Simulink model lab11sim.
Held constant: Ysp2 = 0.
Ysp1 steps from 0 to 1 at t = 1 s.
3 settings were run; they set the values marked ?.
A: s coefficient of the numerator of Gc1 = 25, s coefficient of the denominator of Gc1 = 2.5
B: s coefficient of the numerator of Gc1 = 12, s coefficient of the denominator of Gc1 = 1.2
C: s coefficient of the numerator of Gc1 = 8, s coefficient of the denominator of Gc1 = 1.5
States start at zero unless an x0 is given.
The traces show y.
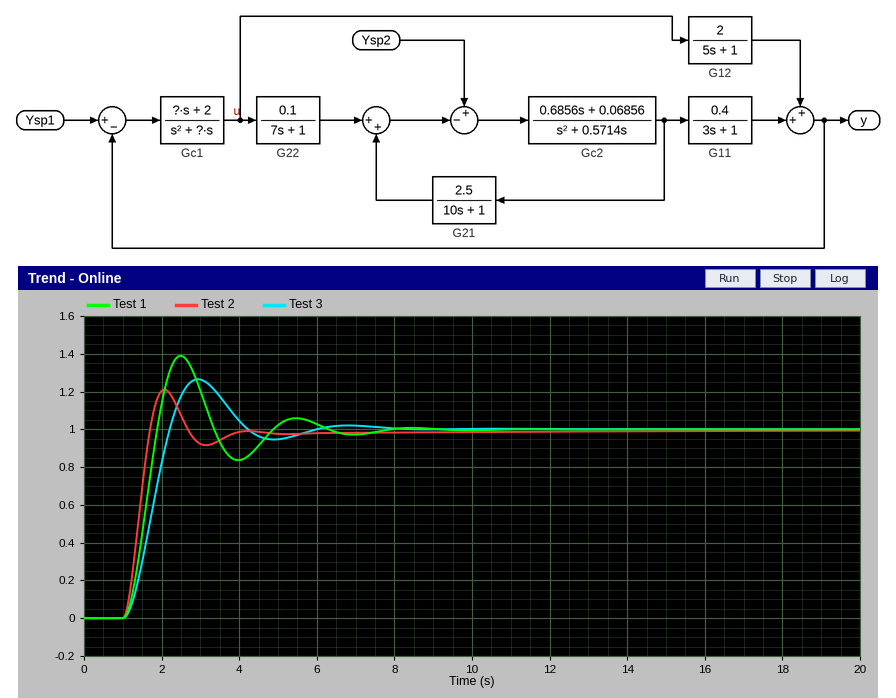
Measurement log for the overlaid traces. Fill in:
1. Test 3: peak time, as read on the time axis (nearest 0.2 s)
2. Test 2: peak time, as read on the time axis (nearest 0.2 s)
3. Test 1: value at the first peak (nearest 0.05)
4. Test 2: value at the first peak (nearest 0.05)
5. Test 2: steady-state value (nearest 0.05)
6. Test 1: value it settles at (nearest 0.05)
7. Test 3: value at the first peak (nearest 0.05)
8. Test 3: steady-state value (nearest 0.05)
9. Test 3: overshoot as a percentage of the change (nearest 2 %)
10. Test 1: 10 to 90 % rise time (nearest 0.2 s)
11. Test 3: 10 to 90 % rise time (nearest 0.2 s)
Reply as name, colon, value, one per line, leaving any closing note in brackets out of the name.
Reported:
Test 3: peak time, as read on the time axis: 3.0 s
Test 2: peak time, as read on the time axis: 2.0 s
Test 1: value at the first peak: 1.40
Test 2: value at the first peak: 1.20
Test 2: steady-state value: 1.00
Test 1: value it settles at: 1.00
Test 3: value at the first peak: 1.25
Test 3: steady-state value: 1.00
Test 3: overshoot as a percentage of the change: 26 %
Test 1: 10 to 90 % rise time: 0.6 s
Test 3: 10 to 90 % rise time: 0.8 s
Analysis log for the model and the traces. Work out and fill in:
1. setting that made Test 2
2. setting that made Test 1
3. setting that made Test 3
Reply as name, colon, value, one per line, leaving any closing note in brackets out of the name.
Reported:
setting that made Test 2: A
setting that made Test 1: B
setting that made Test 3: C
